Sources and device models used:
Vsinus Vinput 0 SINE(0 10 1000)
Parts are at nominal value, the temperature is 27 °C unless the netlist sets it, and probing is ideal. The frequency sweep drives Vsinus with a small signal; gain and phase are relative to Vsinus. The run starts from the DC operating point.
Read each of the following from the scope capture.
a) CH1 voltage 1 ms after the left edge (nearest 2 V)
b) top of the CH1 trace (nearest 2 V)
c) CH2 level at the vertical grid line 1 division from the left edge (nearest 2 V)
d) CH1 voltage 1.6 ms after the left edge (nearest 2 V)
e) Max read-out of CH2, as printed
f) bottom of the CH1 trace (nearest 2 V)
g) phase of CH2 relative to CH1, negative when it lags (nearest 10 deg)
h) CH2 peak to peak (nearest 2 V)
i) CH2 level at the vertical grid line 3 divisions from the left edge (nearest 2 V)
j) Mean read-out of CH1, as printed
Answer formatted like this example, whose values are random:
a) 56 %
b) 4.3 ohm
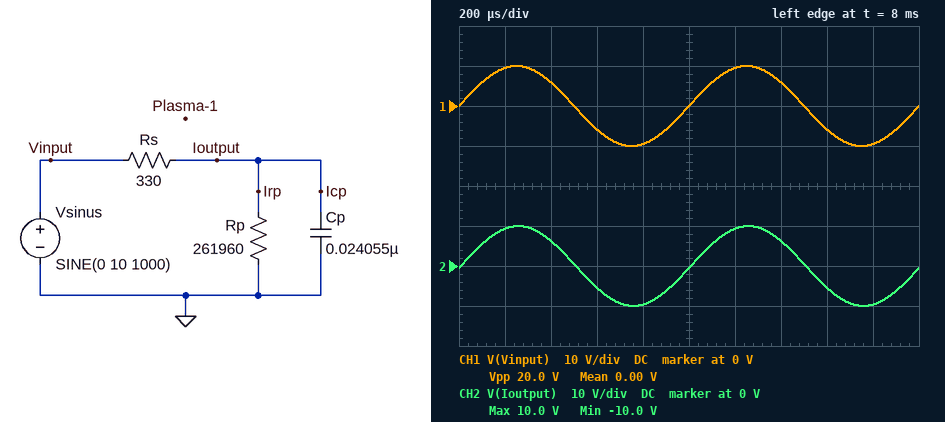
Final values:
a) 0 V
b) 10 V
c) 10 V
d) -6 V
e) 10.0 V
f) -10 V
g) 0 deg
h) 20 V
i) -6 V
j) 0.00 V
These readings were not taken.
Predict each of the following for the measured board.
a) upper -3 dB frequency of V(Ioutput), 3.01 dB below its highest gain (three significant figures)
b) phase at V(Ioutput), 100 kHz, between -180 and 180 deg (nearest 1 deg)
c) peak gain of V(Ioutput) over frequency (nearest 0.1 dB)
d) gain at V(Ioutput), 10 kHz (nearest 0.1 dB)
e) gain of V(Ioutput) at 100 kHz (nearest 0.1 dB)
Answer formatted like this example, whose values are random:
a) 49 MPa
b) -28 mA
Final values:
a) 20.1 kHz
b) -79 deg
c) 0 dB
d) -1.0 dB
e) -14.1 dB
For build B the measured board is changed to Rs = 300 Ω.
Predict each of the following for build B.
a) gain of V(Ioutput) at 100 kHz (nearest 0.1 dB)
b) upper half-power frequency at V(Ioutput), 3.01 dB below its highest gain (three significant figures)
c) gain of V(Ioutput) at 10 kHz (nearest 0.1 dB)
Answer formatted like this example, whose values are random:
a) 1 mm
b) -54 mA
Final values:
a) -13.3 dB
b) 22.1 kHz
c) -0.8 dB
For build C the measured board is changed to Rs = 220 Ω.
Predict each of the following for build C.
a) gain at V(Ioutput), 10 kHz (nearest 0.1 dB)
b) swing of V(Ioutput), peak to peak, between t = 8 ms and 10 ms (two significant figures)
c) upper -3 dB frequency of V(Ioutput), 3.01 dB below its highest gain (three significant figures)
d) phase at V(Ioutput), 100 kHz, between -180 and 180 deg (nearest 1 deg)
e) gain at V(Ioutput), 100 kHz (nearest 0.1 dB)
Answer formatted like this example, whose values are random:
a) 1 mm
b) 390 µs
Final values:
a) -0.5 dB
b) 20 V
c) 30.1 kHz
d) -73 deg
e) -10.8 dB
